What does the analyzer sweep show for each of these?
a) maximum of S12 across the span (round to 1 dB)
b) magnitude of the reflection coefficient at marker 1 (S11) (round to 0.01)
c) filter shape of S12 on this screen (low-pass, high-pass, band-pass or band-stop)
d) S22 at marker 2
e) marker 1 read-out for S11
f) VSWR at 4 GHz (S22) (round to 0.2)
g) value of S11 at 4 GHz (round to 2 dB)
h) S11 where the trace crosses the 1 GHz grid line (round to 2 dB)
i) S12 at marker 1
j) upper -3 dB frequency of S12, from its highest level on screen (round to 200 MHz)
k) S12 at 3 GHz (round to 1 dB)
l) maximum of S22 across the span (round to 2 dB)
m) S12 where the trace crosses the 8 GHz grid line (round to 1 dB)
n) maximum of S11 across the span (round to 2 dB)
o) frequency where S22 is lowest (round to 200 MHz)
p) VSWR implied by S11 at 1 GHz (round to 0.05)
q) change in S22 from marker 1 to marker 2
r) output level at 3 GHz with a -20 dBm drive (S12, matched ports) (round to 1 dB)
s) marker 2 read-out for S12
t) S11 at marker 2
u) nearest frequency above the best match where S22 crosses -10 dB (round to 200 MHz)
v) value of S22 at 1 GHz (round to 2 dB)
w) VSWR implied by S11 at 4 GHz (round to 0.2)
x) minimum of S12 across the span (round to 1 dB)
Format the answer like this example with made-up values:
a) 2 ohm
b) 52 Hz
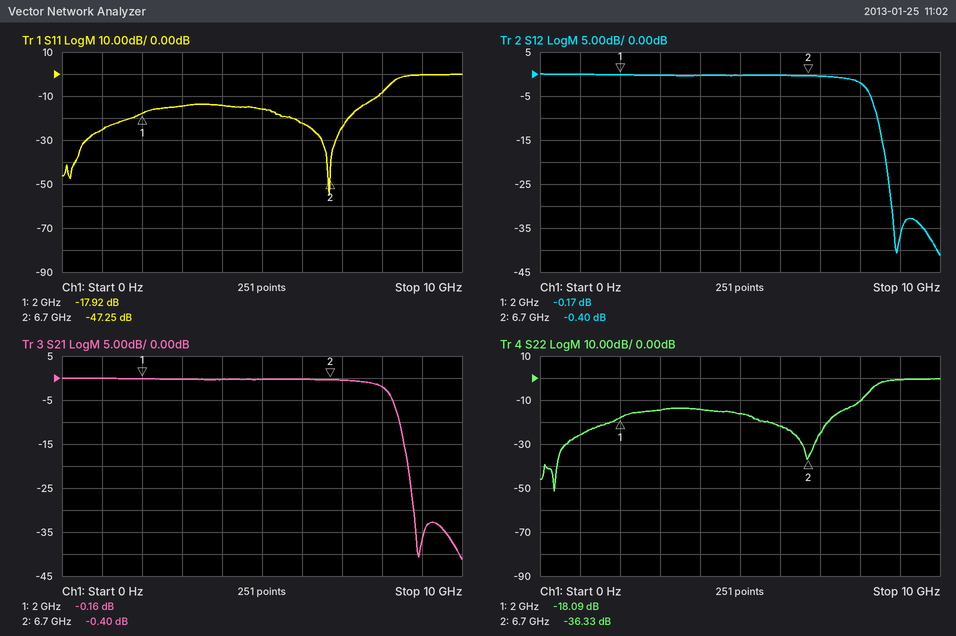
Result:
a) 0 dB
b) 0.13
c) low-pass
d) -36.33 dB
e) -17.92 dB
f) 1.4
g) -14 dB
h) -26 dB
i) -0.17 dB
j) 8.2 GHz
k) 0 dB
l) 0 dB
m) -2 dB
n) 0 dB
o) 400 MHz
p) 1.10
q) -18.24 dB
r) -20 dBm
s) -0.40 dB
t) -47.25 dB
u) 8.0 GHz
v) -26 dB
w) 1.4
x) -41 dB
